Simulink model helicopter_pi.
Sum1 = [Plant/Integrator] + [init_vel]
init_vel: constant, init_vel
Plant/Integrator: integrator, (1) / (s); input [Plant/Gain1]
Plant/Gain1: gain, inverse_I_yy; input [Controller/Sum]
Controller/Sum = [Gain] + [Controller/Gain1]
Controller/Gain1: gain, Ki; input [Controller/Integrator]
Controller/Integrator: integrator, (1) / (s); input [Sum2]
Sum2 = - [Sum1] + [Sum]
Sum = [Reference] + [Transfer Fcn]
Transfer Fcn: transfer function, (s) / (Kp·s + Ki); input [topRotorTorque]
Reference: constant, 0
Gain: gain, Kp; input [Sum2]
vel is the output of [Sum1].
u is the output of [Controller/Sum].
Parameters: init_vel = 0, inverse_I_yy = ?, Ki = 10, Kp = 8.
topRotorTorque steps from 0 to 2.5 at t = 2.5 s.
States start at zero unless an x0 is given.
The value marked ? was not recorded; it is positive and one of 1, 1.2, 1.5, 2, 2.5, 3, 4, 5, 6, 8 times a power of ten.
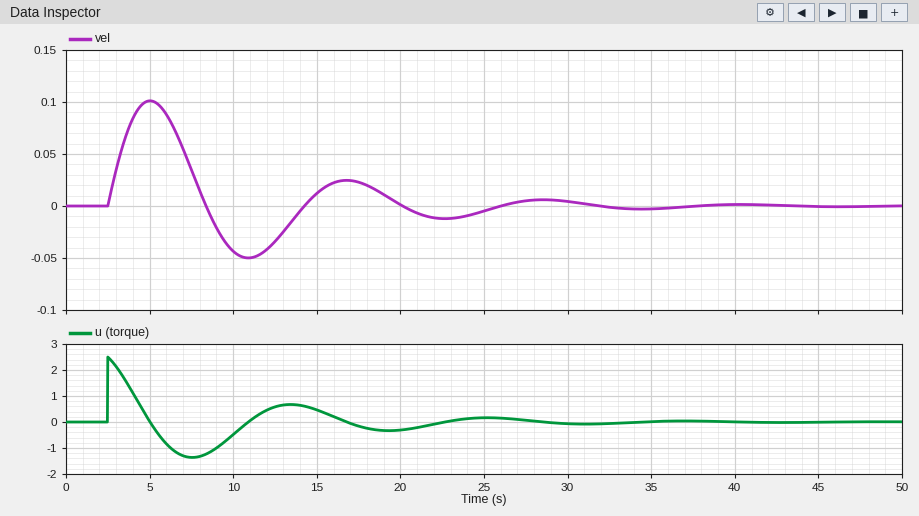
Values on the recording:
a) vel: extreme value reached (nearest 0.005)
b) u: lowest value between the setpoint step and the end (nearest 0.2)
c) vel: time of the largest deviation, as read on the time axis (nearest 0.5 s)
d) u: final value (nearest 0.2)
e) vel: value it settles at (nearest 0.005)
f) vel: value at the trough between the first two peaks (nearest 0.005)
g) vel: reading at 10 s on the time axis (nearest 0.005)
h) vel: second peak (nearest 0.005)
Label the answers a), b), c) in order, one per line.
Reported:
a) 0.100
b) -1.4
c) 5.0 s
d) 0.0
e) 0.000
f) -0.050
g) -0.045
h) 0.025
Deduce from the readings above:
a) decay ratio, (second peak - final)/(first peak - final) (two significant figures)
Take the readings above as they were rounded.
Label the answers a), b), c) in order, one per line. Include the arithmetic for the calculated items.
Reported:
a) (0.025 - 0) / (0.1 - 0) = 0.25
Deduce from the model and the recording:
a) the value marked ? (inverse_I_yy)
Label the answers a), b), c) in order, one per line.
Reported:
a) 0.03
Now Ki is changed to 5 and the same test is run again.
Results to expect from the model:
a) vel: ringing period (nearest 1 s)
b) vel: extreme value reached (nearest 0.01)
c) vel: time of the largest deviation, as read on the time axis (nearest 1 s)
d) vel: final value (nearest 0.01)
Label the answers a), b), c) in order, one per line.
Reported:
a) 17 s
b) 0.13
c) 6 s
d) 0.00
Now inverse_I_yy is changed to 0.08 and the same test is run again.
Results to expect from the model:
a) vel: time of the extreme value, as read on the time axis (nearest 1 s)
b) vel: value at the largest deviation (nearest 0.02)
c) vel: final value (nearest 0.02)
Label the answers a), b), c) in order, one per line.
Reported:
a) 4 s
b) 0.14
c) 0.00
